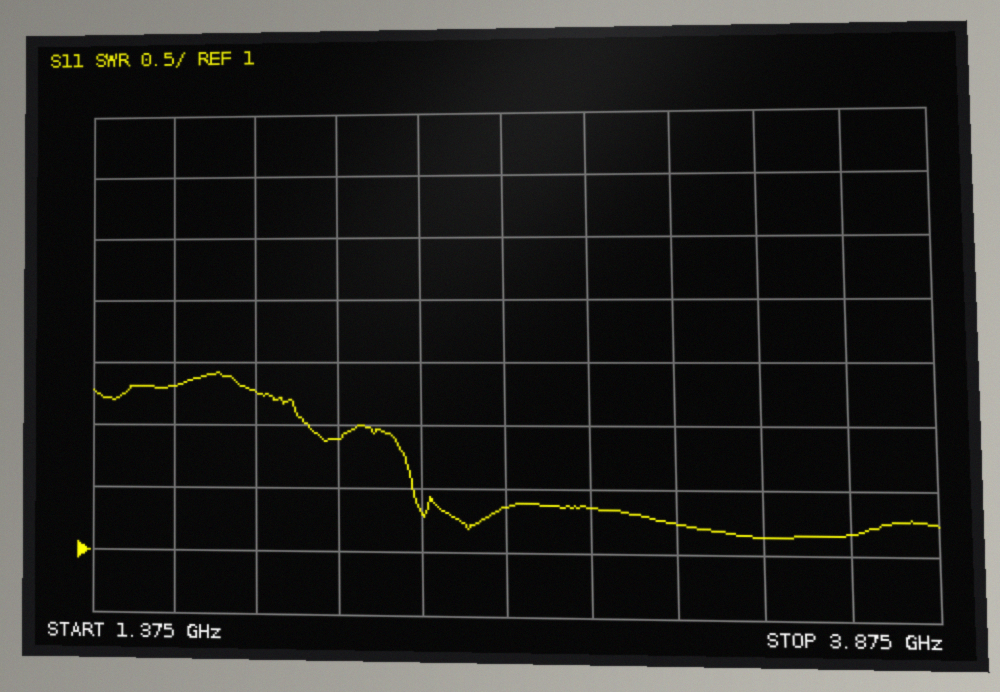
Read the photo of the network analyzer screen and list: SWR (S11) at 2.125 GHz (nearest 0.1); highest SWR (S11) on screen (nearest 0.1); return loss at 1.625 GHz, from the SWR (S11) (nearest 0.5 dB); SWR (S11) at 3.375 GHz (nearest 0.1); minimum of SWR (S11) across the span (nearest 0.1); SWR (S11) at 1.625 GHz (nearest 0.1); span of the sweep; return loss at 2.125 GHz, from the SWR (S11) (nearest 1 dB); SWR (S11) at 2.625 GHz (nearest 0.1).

1.9
2.4
8.0 dB
1.1
1.1
2.3
2.5 GHz
10 dB
1.4
